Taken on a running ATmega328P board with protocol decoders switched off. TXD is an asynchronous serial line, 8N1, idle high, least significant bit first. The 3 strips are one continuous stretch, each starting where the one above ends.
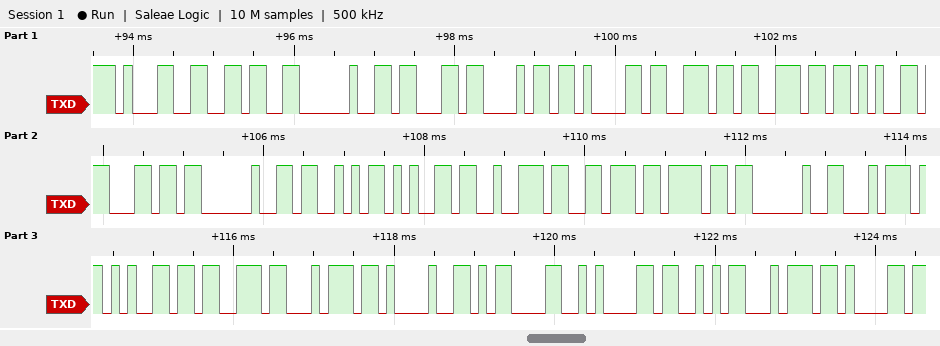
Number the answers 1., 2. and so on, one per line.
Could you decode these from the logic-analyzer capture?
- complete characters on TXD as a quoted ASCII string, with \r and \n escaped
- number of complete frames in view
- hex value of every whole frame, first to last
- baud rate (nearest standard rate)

1. "16 channel Servo test!\r\nSta"
2. 27
3. 31 36 20 63 68 61 6E 6E 65 6C 20 53 65 72 76 6F 20 74 65 73 74 21 0D 0A 53 74 61
4. 9600 baud
